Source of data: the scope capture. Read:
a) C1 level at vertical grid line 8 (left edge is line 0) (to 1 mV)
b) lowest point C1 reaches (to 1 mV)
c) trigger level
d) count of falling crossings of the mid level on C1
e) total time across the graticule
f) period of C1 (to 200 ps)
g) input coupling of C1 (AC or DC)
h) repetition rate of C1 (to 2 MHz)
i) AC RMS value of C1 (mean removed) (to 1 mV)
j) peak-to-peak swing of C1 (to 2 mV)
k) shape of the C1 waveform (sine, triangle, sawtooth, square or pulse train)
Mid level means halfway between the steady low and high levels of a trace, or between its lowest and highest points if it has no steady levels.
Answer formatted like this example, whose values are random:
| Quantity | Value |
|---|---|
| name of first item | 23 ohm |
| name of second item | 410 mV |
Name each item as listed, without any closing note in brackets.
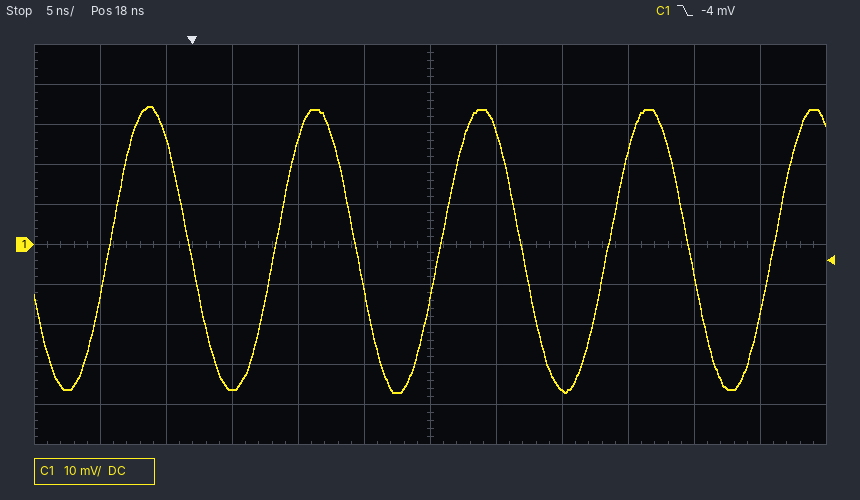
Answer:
| Quantity | Value |
|---|---|
| C1 level at vertical grid line 8 (left edge is line 0) | -36 mV |
| lowest point C1 reaches | -37 mV |
| trigger level | -4 mV |
| count of falling crossings of the mid level on C1 | 4 |
| total time across the graticule | 60 ns |
| period of C1 | 12.6 ns |
| input coupling of C1 | DC |
| repetition rate of C1 | 80 MHz |
| AC RMS value of C1 (mean removed) | 25 mV |
| peak-to-peak swing of C1 | 72 mV |
| shape of the C1 waveform | sine |
